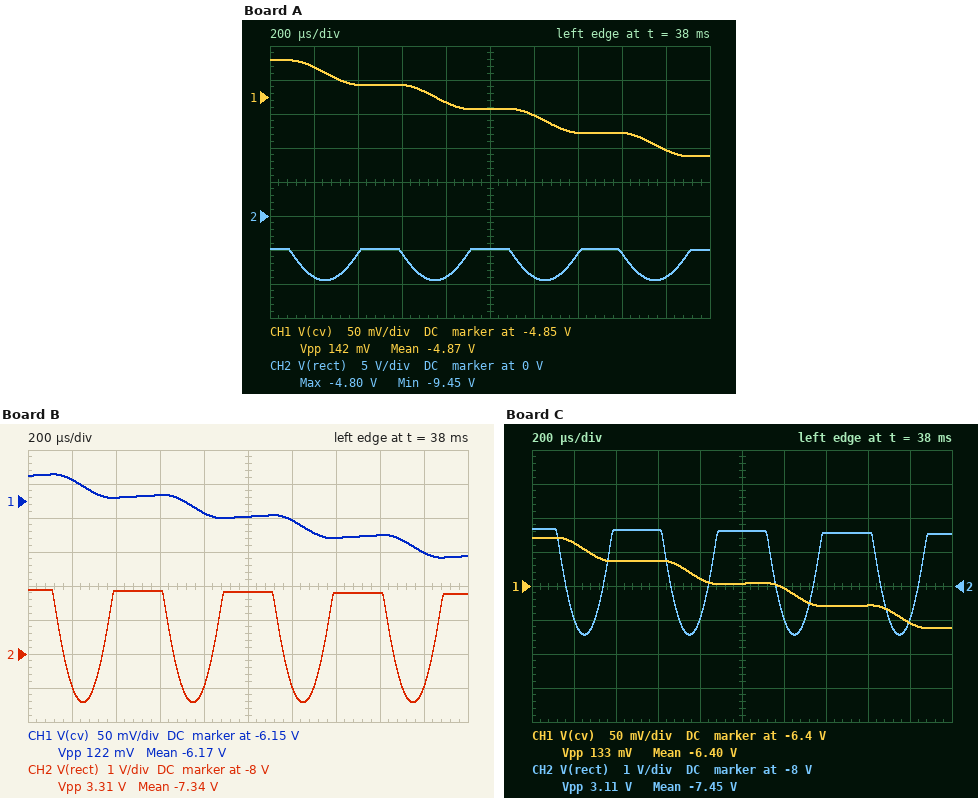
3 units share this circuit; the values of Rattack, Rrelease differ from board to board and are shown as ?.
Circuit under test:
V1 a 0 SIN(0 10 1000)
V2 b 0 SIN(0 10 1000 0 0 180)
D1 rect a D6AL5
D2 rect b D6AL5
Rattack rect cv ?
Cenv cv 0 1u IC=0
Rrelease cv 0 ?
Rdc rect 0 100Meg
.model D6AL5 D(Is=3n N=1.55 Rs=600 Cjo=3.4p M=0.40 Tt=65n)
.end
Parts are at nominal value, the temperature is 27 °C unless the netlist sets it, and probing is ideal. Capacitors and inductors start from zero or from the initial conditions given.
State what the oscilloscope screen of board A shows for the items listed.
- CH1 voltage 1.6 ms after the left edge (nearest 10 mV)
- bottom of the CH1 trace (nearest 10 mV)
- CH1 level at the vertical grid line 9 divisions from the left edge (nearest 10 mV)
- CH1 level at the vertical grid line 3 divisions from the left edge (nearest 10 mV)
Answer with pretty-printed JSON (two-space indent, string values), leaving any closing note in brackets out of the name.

{
  "CH1 voltage 1.6 ms after the left edge": "-4.90 V",
  "bottom of the CH1 trace": "-4.94 V",
  "CH1 level at the vertical grid line 9 divisions from the left edge": "-4.93 V",
  "CH1 level at the vertical grid line 3 divisions from the left edge": "-4.83 V"
}
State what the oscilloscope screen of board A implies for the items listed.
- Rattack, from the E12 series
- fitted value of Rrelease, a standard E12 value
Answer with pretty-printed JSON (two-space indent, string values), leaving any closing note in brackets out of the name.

{
  "Rattack, from the E12 series": "27 kΩ",
  "fitted value of Rrelease, a standard E12 value": "2.7 MΩ"
}
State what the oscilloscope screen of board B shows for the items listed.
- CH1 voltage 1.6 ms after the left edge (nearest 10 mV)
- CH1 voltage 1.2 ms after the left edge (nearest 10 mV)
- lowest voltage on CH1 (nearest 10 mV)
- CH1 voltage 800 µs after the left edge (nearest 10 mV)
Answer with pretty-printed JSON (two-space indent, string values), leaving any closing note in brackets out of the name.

{
  "CH1 voltage 1.6 ms after the left edge": "-6.20 V",
  "CH1 voltage 1.2 ms after the left edge": "-6.18 V",
  "lowest voltage on CH1": "-6.23 V",
  "CH1 voltage 800 µs after the left edge": "-6.17 V"
}
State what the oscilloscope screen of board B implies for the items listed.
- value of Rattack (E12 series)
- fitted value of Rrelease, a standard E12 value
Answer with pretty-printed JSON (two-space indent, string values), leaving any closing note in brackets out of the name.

{
  "value of Rattack": "15 kΩ",
  "fitted value of Rrelease, a standard E12 value": "330 kΩ"
}
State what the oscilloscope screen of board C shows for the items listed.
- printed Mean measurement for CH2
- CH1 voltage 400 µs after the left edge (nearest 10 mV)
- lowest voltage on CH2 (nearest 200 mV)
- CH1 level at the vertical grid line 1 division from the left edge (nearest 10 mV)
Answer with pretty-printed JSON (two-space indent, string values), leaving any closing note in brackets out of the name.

{
  "printed Mean measurement for CH2": "-7.45 V",
  "CH1 voltage 400 µs after the left edge": "-6.36 V",
  "lowest voltage on CH2": "-9.4 V",
  "CH1 level at the vertical grid line 1 division from the left edge": "-6.34 V"
}
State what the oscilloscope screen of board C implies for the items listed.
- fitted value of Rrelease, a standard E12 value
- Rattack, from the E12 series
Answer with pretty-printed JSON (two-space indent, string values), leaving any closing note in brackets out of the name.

{
  "fitted value of Rrelease, a standard E12 value": "1.5 MΩ",
  "Rattack, from the E12 series": "15 kΩ"
}
